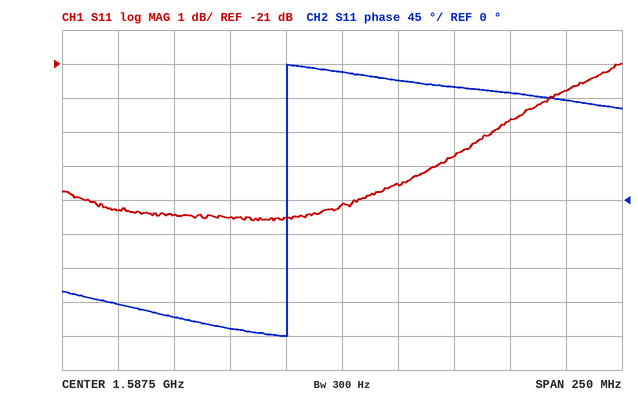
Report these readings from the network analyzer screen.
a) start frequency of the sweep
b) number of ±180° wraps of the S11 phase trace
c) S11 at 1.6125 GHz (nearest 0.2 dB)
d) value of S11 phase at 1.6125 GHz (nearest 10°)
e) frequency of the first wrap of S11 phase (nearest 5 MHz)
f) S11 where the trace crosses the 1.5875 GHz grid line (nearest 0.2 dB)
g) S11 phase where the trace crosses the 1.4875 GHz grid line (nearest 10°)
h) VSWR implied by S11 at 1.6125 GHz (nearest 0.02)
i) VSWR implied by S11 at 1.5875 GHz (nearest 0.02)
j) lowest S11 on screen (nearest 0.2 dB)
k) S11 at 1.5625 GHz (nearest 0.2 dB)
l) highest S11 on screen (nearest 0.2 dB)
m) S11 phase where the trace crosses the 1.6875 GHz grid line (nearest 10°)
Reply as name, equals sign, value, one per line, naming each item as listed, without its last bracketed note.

start frequency of the sweep = 1.4625 GHz
number of ±180° wraps of the S11 phase trace = 1
S11 at 1.6125 GHz = -24.6 dB
value of S11 phase at 1.6125 GHz = 160°
frequency of the first wrap of S11 phase = 1.565 GHz
S11 where the trace crosses the 1.5875 GHz grid line = -25.2 dB
S11 phase where the trace crosses the 1.4875 GHz grid line = -140°
VSWR implied by S11 at 1.6125 GHz = 1.12
VSWR implied by S11 at 1.5875 GHz = 1.12
lowest S11 on screen = -25.6 dB
S11 at 1.5625 GHz = -25.6 dB
highest S11 on screen = -21.0 dB
S11 phase where the trace crosses the 1.6875 GHz grid line = 130°
